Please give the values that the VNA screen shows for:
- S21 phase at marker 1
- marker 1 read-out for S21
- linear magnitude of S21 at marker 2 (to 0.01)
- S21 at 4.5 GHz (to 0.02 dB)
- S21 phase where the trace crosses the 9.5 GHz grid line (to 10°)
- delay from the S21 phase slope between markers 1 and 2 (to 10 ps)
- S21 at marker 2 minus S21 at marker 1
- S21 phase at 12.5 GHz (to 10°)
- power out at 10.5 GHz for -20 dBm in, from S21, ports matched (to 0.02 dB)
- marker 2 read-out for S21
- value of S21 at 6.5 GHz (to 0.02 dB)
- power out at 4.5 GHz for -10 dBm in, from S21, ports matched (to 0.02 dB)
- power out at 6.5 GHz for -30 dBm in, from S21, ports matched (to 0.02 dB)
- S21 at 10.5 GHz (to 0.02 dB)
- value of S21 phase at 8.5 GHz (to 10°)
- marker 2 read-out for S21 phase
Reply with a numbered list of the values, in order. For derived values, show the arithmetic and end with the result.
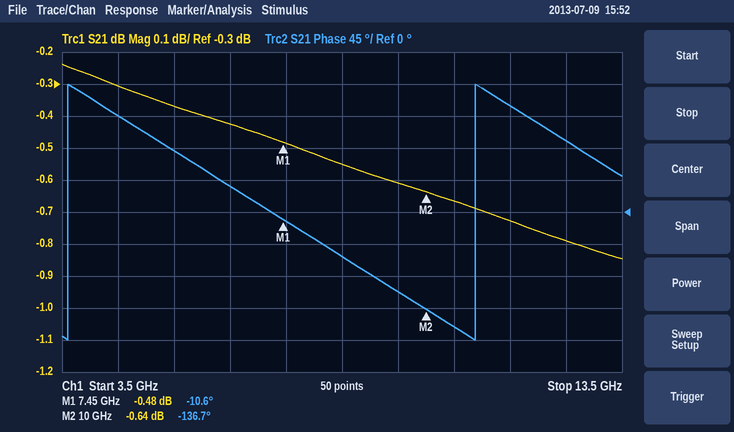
1. -10.6°
2. -0.48 dB
3. 10^(-0.64/20) ≈ 0.93
4. -0.30 dB
5. -110°
6. −(-136.7° − (-10.6°))/(360° × 2.55 GHz) ≈ 137 ps, so 140 ps to the nearest 10 ps
7. -0.64 − (-0.48) = -0.16 dB
8. 100°
9. -20 dBm + (-0.66 dB) = -20.66 dBm
10. -0.64 dB
11. -0.42 dB
12. -10 dBm + (-0.30 dB) = -10.30 dBm
13. -30 dBm + (-0.42 dB) = -30.42 dBm
14. -0.66 dB
15. -60°
16. -136.7°
